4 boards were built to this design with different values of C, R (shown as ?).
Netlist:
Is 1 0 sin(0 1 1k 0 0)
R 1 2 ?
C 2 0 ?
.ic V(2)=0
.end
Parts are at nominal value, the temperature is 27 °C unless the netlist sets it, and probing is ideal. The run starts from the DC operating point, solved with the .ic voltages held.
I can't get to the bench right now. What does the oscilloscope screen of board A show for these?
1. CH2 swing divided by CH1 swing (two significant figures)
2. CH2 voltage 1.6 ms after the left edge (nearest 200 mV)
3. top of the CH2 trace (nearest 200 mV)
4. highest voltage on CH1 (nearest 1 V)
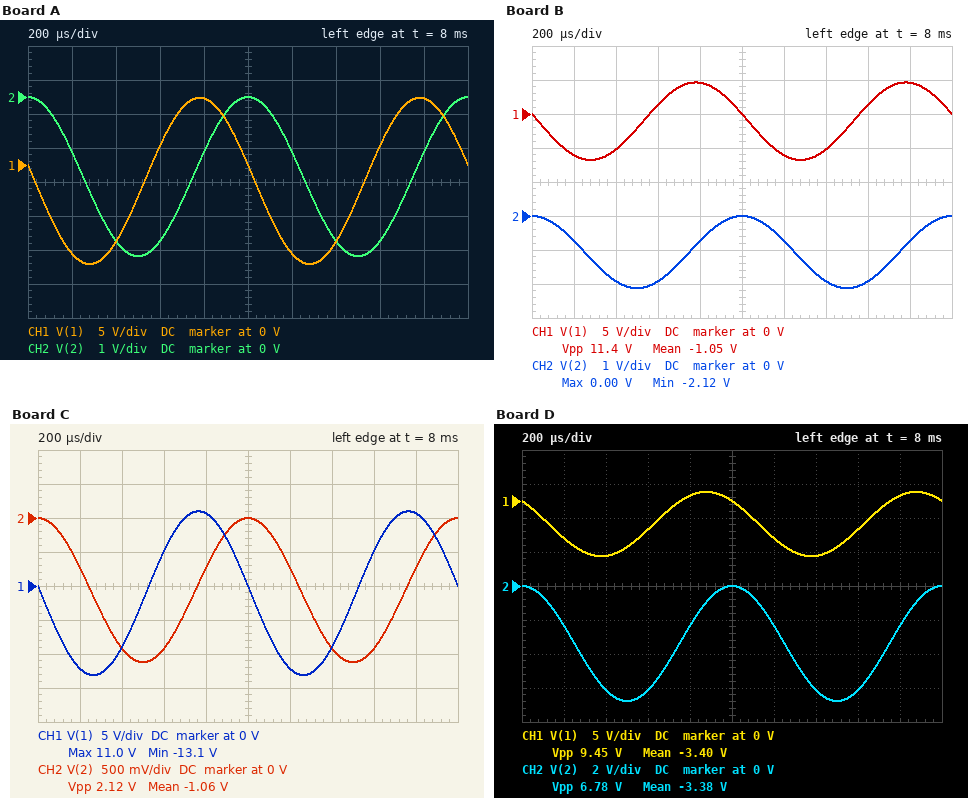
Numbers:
0.19
-4.2 V
0 V
10 V
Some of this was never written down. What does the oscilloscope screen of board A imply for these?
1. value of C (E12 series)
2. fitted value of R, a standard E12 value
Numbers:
68 µF
12 Ω
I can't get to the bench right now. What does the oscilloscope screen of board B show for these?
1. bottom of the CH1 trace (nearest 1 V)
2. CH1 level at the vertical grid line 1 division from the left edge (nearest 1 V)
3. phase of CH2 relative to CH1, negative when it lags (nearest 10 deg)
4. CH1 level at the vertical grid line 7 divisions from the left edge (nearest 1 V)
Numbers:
-7 V
-6 V
-80 deg
-5 V
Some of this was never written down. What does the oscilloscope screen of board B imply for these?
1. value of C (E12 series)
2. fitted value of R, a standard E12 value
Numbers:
150 µF
5.6 Ω
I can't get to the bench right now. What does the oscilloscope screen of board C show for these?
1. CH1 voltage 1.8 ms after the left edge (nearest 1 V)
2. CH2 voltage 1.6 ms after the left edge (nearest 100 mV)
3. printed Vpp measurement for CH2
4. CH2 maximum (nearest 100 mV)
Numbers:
11 V
-1.9 V
2.12 V
0 V
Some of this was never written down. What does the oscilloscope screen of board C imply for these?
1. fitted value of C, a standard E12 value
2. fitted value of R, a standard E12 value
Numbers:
150 µF
12 Ω
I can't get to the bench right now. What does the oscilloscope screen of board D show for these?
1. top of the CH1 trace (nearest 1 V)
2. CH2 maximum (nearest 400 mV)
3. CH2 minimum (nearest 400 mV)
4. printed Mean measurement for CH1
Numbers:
1 V
0 V
-6.8 V
-3.40 V
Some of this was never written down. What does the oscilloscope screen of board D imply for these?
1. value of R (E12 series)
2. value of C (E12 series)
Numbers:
3.3 Ω
47 µF
